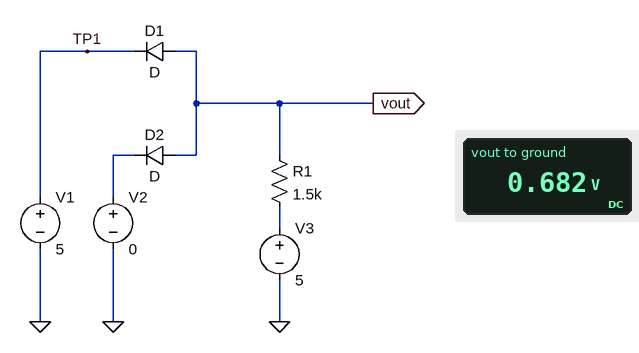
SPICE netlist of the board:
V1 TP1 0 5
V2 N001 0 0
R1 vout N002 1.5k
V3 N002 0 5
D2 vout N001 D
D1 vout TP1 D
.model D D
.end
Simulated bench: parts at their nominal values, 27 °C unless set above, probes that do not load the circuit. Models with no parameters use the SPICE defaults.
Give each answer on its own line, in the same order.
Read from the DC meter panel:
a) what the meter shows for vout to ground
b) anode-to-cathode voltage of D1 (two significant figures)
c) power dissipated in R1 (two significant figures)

0.682 V
-4.3 V
12 mW
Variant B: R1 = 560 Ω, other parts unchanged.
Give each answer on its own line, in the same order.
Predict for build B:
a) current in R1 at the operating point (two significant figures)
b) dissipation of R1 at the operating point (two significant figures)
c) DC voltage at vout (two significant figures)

7.7 mA
33 mW
710 mV
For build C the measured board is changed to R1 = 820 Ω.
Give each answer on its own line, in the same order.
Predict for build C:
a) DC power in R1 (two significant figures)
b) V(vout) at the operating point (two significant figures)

23 mW
700 mV
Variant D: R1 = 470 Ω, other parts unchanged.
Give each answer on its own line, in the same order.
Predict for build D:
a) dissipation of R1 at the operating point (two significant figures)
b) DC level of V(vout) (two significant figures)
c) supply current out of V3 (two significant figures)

39 mW
710 mV
9.1 mA
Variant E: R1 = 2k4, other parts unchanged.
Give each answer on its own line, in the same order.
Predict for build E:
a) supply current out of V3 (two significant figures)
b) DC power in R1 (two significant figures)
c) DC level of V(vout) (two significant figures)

1.8 mA
7.8 mW
670 mV
